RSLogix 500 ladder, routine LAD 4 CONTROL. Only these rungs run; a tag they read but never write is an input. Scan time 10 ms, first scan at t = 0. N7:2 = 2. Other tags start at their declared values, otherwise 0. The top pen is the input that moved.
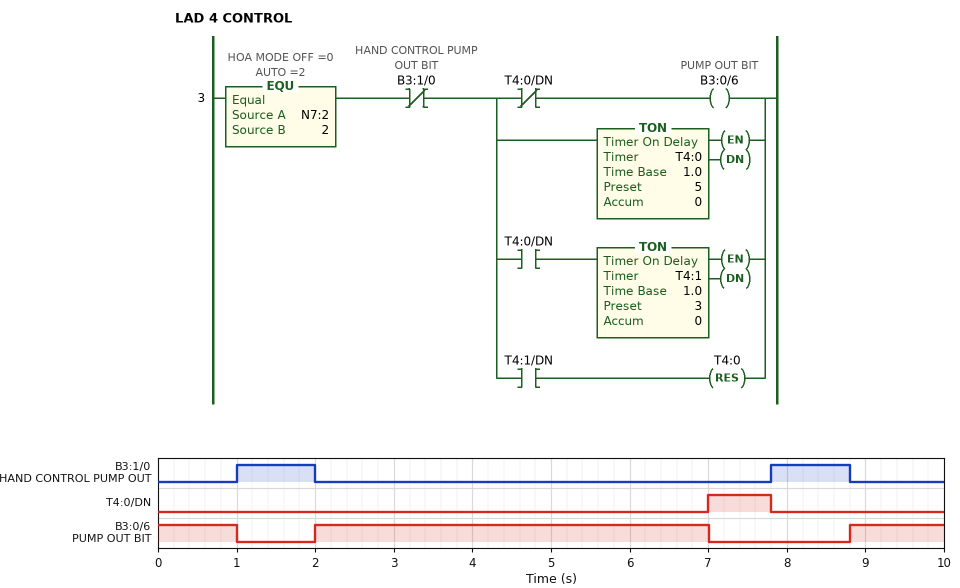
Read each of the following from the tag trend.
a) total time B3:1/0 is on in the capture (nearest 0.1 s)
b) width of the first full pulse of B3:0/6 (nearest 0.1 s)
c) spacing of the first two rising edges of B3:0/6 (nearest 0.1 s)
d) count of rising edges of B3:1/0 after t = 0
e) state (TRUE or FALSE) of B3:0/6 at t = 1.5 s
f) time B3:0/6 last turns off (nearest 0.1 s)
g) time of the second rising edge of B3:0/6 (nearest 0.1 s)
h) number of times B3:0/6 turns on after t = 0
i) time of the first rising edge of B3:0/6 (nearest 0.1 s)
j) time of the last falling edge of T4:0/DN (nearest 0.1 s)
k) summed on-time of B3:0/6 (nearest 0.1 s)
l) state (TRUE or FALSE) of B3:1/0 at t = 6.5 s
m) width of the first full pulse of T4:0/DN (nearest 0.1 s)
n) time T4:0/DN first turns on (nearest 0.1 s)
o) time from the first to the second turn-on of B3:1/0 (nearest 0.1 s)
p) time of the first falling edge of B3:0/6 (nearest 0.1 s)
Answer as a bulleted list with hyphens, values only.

- 2.0 s
- 5.0 s
- 6.8 s
- 2
- FALSE
- 7.0 s
- 8.8 s
- 2
- 2.0 s
- 7.8 s
- 7.2 s
- FALSE
- 0.8 s
- 7.0 s
- 6.8 s
- 1.0 s
